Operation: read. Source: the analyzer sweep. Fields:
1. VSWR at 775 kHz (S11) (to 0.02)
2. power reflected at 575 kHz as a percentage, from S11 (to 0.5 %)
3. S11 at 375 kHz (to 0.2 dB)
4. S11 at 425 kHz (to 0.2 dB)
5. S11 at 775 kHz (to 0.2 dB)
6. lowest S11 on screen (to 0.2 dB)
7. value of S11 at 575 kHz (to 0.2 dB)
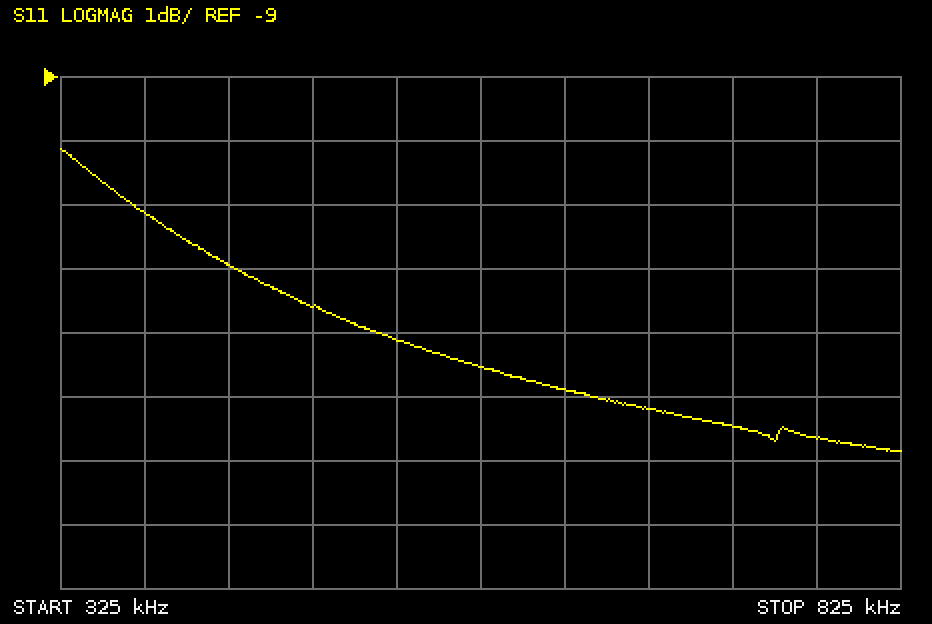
1.46
4.5 %
-11.2 dB
-12.0 dB
-14.6 dB
-14.8 dB
-13.6 dB
